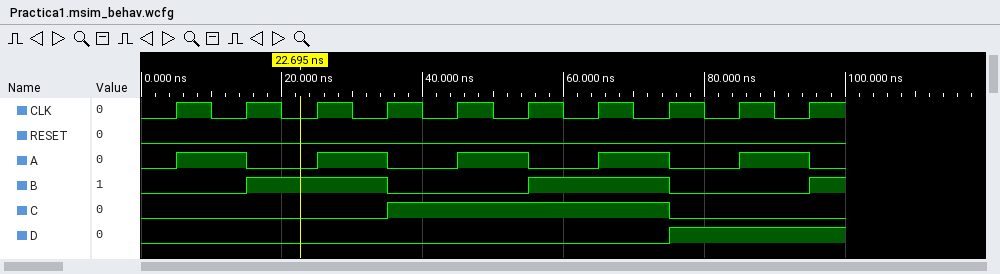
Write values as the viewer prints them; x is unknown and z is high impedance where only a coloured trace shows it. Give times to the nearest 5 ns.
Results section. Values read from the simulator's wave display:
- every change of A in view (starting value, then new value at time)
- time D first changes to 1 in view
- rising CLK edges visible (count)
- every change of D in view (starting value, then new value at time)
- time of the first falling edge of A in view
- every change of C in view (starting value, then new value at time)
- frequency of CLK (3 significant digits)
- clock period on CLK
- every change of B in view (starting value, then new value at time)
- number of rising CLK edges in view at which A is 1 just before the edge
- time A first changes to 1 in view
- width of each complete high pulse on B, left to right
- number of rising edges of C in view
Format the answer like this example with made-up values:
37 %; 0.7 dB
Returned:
0, 1 at 5 ns, 0 at 15 ns, 1 at 25 ns, 0 at 35 ns, 1 at 45 ns, 0 at 55 ns, 1 at 65 ns, 0 at 75 ns, 1 at 85 ns, 0 at 95 ns; 75 ns; 10; 0, 1 at 75 ns; 15 ns; 0, 1 at 35 ns, 0 at 75 ns; 100 MHz; 10 ns; 0, 1 at 15 ns, 0 at 35 ns, 1 at 55 ns, 0 at 75 ns, 1 at 95 ns; 5; 5 ns; 20 ns, 20 ns; 1
